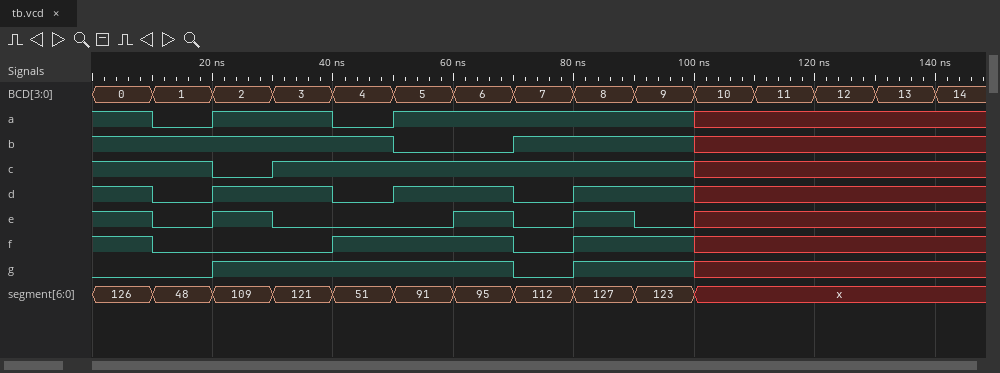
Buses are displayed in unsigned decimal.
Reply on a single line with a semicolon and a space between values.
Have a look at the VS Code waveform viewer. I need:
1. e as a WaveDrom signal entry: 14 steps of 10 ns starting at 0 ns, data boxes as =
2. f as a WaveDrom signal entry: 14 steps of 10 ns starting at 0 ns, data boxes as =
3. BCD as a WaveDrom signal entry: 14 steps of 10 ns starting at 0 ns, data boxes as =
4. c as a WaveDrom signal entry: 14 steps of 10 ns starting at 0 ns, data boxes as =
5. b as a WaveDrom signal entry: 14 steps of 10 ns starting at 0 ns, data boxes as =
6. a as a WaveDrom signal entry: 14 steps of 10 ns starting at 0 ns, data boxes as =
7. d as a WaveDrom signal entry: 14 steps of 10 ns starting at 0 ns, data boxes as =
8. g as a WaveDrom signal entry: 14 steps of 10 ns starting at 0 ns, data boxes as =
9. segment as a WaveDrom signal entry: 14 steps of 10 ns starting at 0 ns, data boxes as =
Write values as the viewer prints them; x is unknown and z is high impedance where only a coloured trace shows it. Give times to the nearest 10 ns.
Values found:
{name: 'e', wave: '1010..1010x...'}; {name: 'f', wave: '10..1..01.x...'}; {name: 'BCD', wave: '==============', data: '0 1 2 3 4 5 6 7 8 9 10 11 12 13'}; {name: 'c', wave: '1.01......x...'}; {name: 'b', wave: '1....0.1..x...'}; {name: 'a', wave: '101.01....x...'}; {name: 'd', wave: '101.01.01.x...'}; {name: 'g', wave: '0.1....01.x...'}; {name: 'segment', wave: '==========x...', data: '126 48 109 121 51 91 95 112 127 123'}
